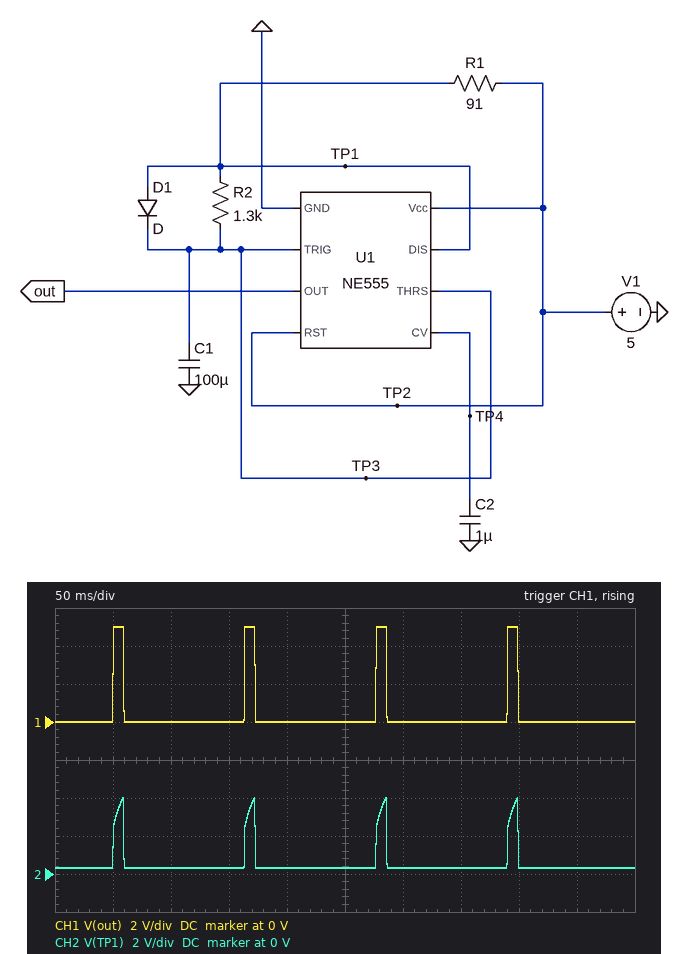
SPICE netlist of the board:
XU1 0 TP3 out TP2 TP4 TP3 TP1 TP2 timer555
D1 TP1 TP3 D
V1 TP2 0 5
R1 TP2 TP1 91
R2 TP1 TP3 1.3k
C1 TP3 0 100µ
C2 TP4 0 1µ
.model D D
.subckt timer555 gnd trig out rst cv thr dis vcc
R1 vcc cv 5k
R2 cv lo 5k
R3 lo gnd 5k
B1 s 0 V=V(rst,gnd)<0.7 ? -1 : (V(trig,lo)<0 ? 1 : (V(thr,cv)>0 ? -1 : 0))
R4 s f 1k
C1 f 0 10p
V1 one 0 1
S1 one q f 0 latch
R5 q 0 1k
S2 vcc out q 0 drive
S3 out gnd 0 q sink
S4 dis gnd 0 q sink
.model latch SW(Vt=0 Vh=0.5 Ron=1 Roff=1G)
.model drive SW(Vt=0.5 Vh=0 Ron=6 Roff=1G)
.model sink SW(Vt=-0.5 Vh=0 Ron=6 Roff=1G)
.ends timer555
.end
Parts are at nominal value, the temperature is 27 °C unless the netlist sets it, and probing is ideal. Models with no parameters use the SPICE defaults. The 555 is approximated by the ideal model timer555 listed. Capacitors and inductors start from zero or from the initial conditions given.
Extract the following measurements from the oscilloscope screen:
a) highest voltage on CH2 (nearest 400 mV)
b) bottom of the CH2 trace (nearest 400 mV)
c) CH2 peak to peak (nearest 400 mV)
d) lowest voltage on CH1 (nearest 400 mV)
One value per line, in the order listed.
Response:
4.0 V
400 mV
3.6 V
0 V
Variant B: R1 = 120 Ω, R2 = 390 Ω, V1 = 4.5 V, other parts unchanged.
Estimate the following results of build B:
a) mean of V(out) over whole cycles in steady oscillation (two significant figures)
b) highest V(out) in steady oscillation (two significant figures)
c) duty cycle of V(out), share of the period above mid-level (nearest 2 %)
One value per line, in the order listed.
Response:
1.3 V
4.5 V
30 %
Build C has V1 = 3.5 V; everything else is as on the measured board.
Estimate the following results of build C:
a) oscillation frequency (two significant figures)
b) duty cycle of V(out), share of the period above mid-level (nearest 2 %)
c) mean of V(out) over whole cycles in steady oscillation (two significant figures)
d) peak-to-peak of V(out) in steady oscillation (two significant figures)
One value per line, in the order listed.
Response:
8.6 Hz
10 %
350 mV
3.5 V
